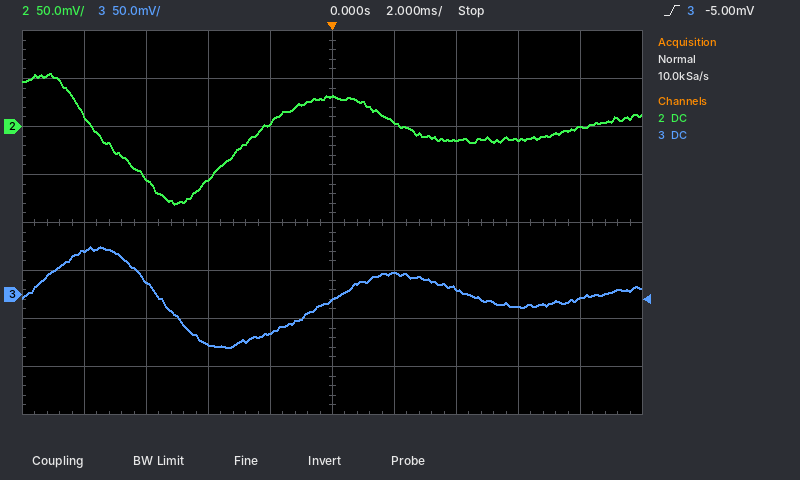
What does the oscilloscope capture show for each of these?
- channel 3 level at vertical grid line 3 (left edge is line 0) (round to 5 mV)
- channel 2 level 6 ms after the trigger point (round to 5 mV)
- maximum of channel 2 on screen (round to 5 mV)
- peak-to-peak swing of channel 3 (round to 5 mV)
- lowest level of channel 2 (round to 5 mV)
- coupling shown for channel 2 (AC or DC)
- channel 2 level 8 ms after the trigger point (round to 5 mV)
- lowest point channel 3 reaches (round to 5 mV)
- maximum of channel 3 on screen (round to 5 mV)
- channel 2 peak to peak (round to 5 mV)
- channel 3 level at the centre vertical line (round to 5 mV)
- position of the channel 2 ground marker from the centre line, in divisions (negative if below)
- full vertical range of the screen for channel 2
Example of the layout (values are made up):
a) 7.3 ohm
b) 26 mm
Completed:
a) -50 mV
b) -15 mV
c) 55 mV
d) 105 mV
e) -80 mV
f) DC
g) 0 mV
h) -55 mV
i) 50 mV
j) 135 mV
k) -5 mV
l) +2.0 div
m) 400 mV
